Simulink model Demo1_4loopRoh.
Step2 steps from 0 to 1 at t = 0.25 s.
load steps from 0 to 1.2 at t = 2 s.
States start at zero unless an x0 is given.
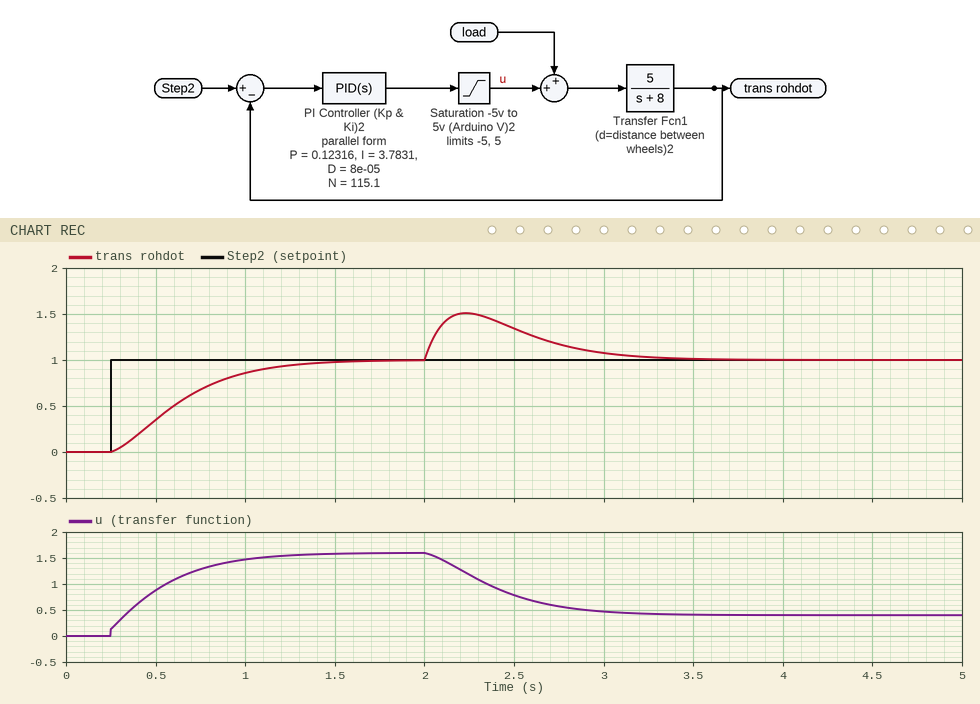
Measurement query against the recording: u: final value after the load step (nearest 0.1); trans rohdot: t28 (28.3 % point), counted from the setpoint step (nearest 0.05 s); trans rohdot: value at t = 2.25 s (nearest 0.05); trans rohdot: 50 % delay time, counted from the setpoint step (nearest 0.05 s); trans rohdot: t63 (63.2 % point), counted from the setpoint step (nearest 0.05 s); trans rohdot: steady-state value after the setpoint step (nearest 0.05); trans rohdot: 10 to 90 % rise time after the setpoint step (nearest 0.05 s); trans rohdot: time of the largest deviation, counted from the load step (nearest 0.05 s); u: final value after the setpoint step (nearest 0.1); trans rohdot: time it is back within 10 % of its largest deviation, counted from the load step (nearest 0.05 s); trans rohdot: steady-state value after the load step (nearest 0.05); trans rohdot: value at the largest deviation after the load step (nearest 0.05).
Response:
0.4
0.20 s
1.50
0.35 s
0.45 s
1.00
0.75 s
0.25 s
1.6
1.10 s
1.00
1.50
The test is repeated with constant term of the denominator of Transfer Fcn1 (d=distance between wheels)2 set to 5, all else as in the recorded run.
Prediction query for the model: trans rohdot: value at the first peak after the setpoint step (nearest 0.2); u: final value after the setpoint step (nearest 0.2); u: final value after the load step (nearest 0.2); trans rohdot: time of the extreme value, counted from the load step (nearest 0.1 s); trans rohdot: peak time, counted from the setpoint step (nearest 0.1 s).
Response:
1.0
1.0
-0.2
0.3 s
0.9 s
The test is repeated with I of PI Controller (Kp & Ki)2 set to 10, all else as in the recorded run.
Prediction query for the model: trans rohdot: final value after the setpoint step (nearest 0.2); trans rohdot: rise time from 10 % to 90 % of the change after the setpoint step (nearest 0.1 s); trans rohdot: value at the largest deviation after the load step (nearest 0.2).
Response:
1.0
0.3 s
1.4
